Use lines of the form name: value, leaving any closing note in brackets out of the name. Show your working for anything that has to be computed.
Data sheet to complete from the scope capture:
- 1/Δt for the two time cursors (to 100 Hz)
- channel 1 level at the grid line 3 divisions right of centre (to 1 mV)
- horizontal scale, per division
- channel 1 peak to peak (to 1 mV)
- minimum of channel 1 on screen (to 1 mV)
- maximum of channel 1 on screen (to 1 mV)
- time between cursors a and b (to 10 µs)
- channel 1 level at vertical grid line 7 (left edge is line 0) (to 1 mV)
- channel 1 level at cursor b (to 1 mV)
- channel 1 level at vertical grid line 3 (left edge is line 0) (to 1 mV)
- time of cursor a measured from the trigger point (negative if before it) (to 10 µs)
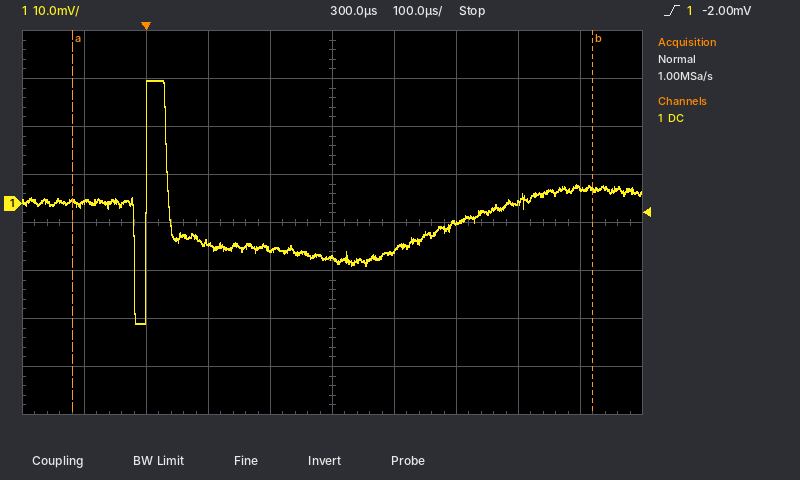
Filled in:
1/Δt for the two time cursors: 1 / 840 µs ≈ 1.2 kHz
channel 1 level at the grid line 3 divisions right of centre: 0 mV
horizontal scale, per division: 100 µs
channel 1 peak to peak: 26 mV − (-25 mV) = 51 mV
minimum of channel 1 on screen: -25 mV
maximum of channel 1 on screen: 26 mV
time between cursors a and b: 840 µs
channel 1 level at vertical grid line 7 (left edge is line 0): -4 mV
channel 1 level at cursor b: 3 mV
channel 1 level at vertical grid line 3 (left edge is line 0): -8 mV
time of cursor a measured from the trigger point (negative if before it): -120 µs
